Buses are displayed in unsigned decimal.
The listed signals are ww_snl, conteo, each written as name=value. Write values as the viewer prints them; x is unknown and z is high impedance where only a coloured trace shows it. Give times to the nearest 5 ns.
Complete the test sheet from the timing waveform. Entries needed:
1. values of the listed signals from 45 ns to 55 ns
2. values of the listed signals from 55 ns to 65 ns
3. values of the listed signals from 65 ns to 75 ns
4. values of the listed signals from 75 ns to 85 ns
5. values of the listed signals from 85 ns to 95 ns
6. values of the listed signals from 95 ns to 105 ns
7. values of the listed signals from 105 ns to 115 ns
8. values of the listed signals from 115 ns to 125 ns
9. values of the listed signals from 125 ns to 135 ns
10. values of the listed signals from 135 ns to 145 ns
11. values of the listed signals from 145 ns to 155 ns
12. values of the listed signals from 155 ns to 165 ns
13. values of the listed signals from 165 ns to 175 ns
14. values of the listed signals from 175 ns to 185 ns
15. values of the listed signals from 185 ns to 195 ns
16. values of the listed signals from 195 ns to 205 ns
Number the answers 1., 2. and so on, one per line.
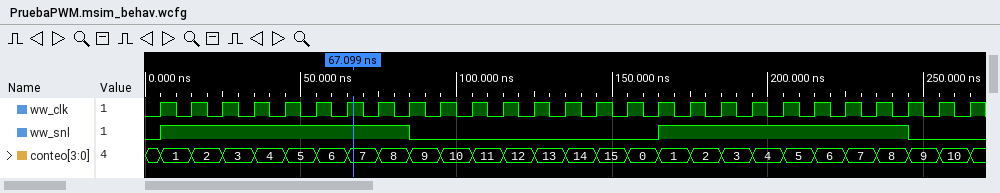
1. ww_snl=1, conteo=5
2. ww_snl=1, conteo=6
3. ww_snl=1, conteo=7
4. ww_snl=1, conteo=8
5. ww_snl=0, conteo=9
6. ww_snl=0, conteo=10
7. ww_snl=0, conteo=11
8. ww_snl=0, conteo=12
9. ww_snl=0, conteo=13
10. ww_snl=0, conteo=14
11. ww_snl=0, conteo=15
12. ww_snl=0, conteo=0
13. ww_snl=1, conteo=1
14. ww_snl=1, conteo=2
15. ww_snl=1, conteo=3
16. ww_snl=1, conteo=4
